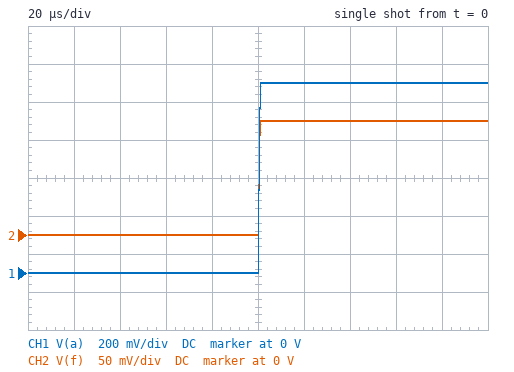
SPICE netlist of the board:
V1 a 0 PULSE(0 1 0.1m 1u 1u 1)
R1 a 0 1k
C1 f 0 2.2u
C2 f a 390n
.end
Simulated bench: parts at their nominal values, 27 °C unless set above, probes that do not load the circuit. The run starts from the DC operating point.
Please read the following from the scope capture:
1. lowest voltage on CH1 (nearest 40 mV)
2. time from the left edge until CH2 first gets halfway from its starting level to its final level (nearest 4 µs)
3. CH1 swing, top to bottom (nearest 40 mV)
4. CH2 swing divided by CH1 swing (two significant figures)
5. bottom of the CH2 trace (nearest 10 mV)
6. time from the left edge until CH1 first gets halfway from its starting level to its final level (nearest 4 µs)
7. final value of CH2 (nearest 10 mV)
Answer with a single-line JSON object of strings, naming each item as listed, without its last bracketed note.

{"lowest voltage on CH1": "0 V", "time from the left edge until CH2 first gets halfway from its starting level to its final level": "100 µs", "CH1 swing, top to bottom": "1.00 V", "CH2 swing divided by CH1 swing": "0.15", "bottom of the CH2 trace": "0 V", "time from the left edge until CH1 first gets halfway from its starting level to its final level": "100 µs", "final value of CH2": "150 mV"}
